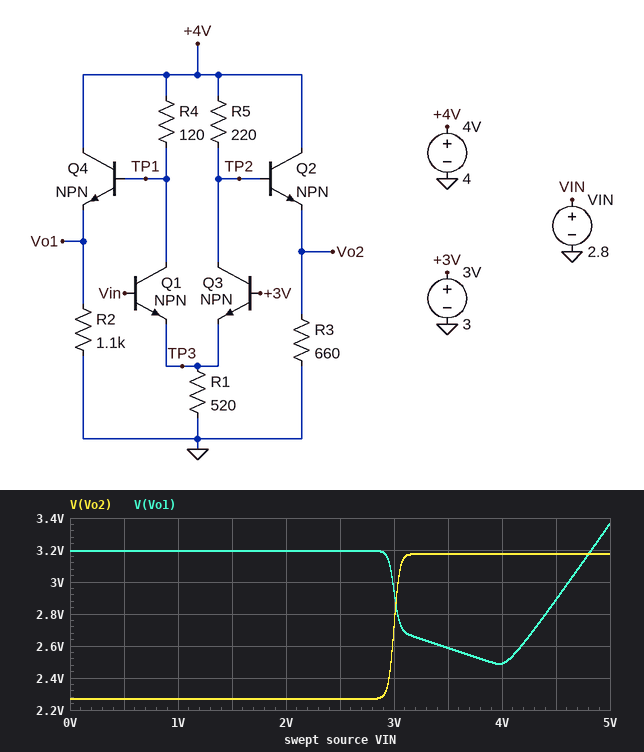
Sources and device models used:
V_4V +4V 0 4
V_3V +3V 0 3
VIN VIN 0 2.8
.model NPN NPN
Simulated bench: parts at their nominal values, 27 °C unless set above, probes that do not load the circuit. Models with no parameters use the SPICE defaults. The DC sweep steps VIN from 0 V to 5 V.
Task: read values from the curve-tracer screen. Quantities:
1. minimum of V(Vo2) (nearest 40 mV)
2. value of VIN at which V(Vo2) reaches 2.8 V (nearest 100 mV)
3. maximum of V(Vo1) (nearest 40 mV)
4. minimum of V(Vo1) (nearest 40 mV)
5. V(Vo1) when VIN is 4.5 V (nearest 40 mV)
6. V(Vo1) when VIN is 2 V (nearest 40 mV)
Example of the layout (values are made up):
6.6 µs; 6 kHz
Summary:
2.28 V; 3.0 V; 3.36 V; 2.48 V; 2.88 V; 3.20 V
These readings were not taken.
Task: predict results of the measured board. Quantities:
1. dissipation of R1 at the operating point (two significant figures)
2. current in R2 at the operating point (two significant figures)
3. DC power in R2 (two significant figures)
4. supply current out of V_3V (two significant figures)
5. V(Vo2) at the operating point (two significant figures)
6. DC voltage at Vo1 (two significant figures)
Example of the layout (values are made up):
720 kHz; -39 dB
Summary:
9.2 mW; 2.9 mA; 9.3 mW; 42 µA; 2.3 V; 3.2 V
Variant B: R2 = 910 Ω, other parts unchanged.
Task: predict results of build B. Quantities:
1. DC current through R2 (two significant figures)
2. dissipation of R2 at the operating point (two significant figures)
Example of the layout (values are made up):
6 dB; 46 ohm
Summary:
3.5 mA; 11 mW
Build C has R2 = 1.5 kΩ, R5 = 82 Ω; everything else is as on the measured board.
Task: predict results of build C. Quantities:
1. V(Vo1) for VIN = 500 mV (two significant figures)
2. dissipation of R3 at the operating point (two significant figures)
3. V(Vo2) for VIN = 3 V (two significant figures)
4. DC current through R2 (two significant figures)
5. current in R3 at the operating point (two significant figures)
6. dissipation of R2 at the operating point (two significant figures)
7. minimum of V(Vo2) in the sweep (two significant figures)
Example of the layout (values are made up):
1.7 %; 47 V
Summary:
3.2 V; 12 mW; 3.0 V; 2.1 mA; 4.3 mA; 6.8 mW; 2.8 V
